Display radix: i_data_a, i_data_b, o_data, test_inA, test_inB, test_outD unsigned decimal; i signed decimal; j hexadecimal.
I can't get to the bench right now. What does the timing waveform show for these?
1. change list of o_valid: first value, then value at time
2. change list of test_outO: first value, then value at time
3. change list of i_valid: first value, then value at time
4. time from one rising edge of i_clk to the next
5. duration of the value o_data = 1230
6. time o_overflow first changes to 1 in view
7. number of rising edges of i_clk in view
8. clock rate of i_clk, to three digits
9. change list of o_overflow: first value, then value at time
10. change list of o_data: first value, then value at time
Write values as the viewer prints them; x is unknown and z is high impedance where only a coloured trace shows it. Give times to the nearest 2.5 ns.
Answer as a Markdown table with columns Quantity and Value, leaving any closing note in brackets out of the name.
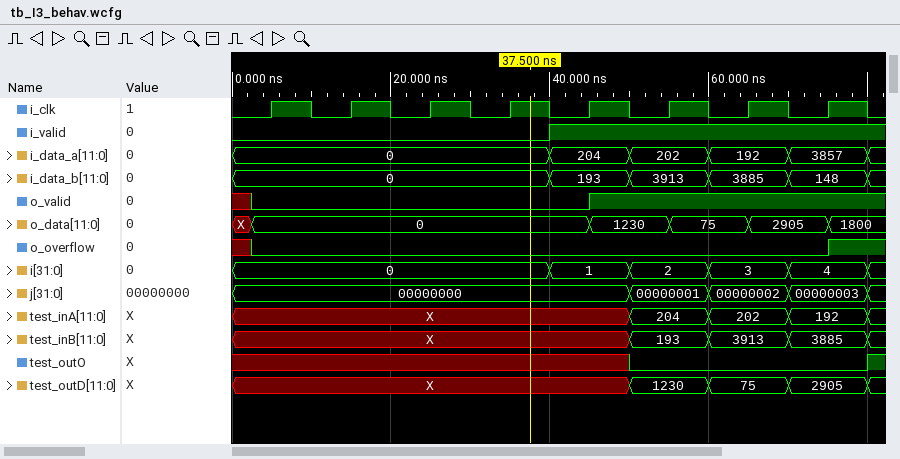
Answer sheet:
| Quantity | Value |
|---|---|
| change list of o_valid: first value, then value at time | x, 0 at 2.5 ns, 1 at 45 ns |
| change list of test_outO: first value, then value at time | x, 0 at 50 ns, 1 at 80 ns |
| change list of i_valid: first value, then value at time | 0, 1 at 40 ns |
| time from one rising edge of i_clk to the next | 10 ns |
| duration of the value o_data = 1230 | 10 ns |
| time o_overflow first changes to 1 in view | 75 ns |
| number of rising edges of i_clk in view | 8 |
| clock rate of i_clk, to three digits | 100 MHz |
| change list of o_overflow: first value, then value at time | x, 0 at 2.5 ns, 1 at 75 ns |
| change list of o_data: first value, then value at time | X, 0 at 2.5 ns, 1230 at 45 ns, 75 at 55 ns, 2905 at 65 ns, 1800 at 75 ns |
